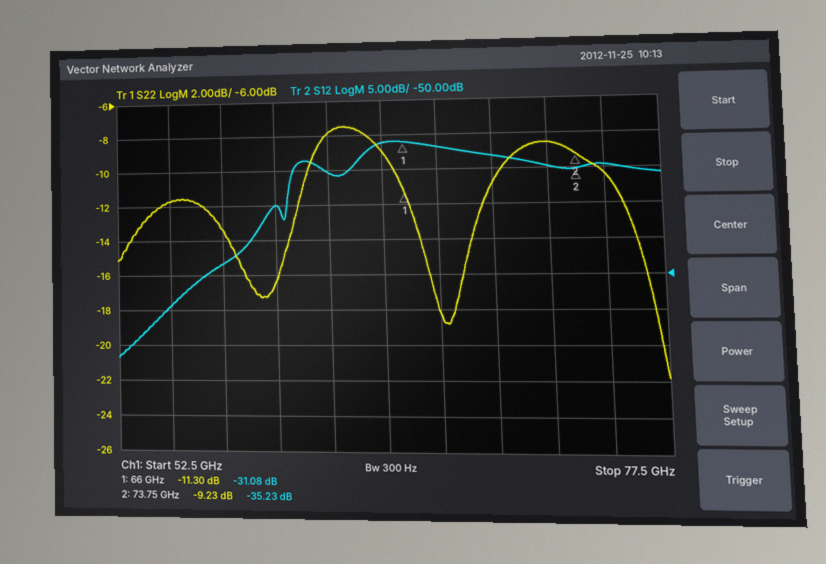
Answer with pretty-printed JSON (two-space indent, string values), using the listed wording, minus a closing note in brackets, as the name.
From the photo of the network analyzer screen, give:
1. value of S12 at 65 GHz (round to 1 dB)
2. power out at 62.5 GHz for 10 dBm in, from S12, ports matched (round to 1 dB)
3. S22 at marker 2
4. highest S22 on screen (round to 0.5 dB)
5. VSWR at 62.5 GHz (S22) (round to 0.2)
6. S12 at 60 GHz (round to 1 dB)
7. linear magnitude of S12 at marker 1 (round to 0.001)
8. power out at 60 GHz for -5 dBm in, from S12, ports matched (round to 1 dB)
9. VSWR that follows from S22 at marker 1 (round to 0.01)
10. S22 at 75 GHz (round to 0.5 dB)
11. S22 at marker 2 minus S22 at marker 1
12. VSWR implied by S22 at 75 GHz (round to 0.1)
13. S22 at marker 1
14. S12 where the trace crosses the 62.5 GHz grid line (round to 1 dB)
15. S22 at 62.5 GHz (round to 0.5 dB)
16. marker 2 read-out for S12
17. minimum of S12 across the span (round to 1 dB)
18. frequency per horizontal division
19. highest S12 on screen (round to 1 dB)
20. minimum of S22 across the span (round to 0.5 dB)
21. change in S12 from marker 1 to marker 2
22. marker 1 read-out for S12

{
  "value of S12 at 65 GHz": "-31 dB",
  "power out at 62.5 GHz for 10 dBm in, from S12, ports matched": "-25 dBm",
  "S22 at marker 2": "-9.23 dB",
  "highest S22 on screen": "-7.5 dB",
  "VSWR at 62.5 GHz (S22)": "2.4",
  "S12 at 60 GHz": "-40 dB",
  "linear magnitude of S12 at marker 1": "0.028",
  "power out at 60 GHz for -5 dBm in, from S12, ports matched": "-45 dBm",
  "VSWR that follows from S22 at marker 1": "1.75",
  "S22 at 75 GHz": "-10.5 dB",
  "S22 at marker 2 minus S22 at marker 1": "2.07 dB",
  "VSWR implied by S22 at 75 GHz": "1.9",
  "S22 at marker 1": "-11.30 dB",
  "S12 where the trace crosses the 62.5 GHz grid line": "-35 dB",
  "S22 at 62.5 GHz": "-8.0 dB",
  "marker 2 read-out for S12": "-35.23 dB",
  "minimum of S12 across the span": "-62 dB",
  "frequency per horizontal division": "2.5 GHz",
  "highest S12 on screen": "-31 dB",
  "minimum of S22 across the span": "-22.0 dB",
  "change in S12 from marker 1 to marker 2": "-4.15 dB",
  "marker 1 read-out for S12": "-31.08 dB"
}
